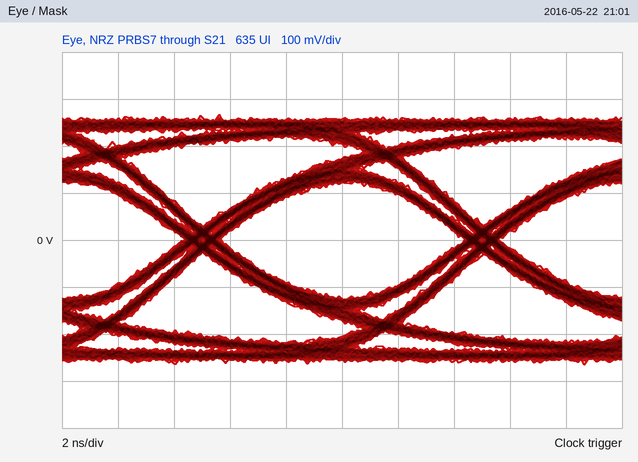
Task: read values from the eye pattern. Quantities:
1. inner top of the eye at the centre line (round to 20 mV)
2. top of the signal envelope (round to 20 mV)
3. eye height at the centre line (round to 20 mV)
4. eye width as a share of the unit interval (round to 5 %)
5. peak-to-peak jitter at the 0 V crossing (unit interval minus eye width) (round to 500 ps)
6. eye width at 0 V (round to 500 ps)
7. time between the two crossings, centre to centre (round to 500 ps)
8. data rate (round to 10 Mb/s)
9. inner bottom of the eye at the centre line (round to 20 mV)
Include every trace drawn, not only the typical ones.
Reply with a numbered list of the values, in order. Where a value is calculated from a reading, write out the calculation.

1. 120 mV
2. 260 mV
3. 240 mV
4. 8.5 ns / 10.0 ns ≈ 85 %
5. 1.5 ns
6. 8.5 ns
7. 10.0 ns
8. 100 Mb/s
9. -120 mV
